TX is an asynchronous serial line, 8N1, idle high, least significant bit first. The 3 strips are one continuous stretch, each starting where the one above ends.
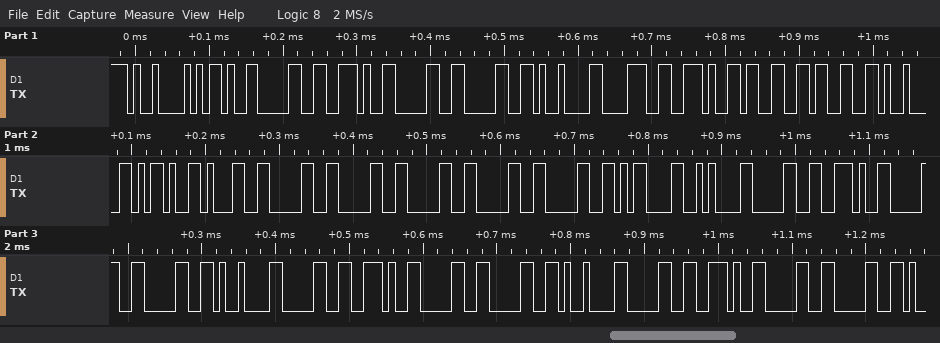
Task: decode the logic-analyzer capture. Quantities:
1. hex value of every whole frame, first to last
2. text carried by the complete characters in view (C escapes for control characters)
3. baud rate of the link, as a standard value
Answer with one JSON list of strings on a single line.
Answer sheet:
["09 2D 30 2E 30 30 09 38 2E 33 33 09 2D 31 30 30 30 30 30 0D 0A 30 2E 30 30 09 30 2E 30 30 09 30 2E 30 30", "\"\\t-0.00\\t8.33\\t-100000\\r\\n0.00\\t0.00\\t0.00\"", "115200 baud"]
